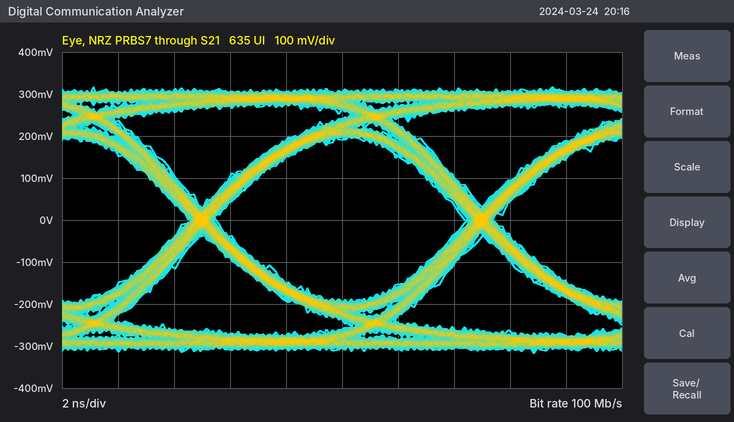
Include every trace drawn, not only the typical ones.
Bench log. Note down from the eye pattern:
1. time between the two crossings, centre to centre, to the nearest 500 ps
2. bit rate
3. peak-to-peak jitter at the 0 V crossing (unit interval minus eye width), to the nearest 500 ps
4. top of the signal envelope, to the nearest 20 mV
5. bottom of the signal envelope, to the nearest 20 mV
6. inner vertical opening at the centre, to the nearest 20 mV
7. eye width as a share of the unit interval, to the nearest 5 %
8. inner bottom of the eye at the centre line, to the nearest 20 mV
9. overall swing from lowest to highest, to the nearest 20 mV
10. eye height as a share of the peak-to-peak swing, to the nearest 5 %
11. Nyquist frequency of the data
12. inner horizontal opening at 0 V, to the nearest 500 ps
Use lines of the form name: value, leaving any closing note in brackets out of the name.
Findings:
time between the two crossings, centre to centre, to the nearest 500 ps: 10.0 ns
bit rate: 100 Mb/s
peak-to-peak jitter at the 0 V crossing (unit interval minus eye width), to the nearest 500 ps: 1.0 ns
top of the signal envelope, to the nearest 20 mV: 320 mV
bottom of the signal envelope, to the nearest 20 mV: -320 mV
inner vertical opening at the centre, to the nearest 20 mV: 380 mV
eye width as a share of the unit interval, to the nearest 5 %: 90 %
inner bottom of the eye at the centre line, to the nearest 20 mV: -200 mV
overall swing from lowest to highest, to the nearest 20 mV: 640 mV
eye height as a share of the peak-to-peak swing, to the nearest 5 %: 60 %
Nyquist frequency of the data: 50 MHz
inner horizontal opening at 0 V, to the nearest 500 ps: 9.0 ns
